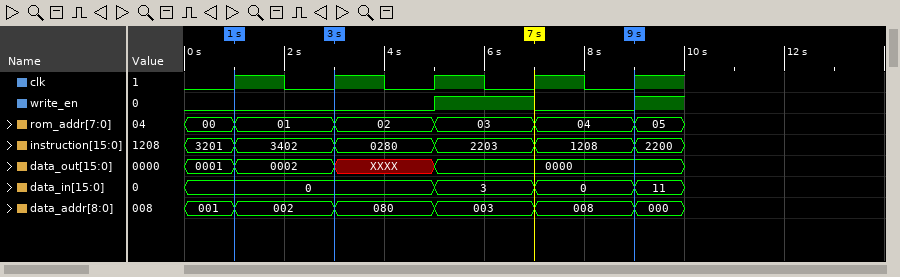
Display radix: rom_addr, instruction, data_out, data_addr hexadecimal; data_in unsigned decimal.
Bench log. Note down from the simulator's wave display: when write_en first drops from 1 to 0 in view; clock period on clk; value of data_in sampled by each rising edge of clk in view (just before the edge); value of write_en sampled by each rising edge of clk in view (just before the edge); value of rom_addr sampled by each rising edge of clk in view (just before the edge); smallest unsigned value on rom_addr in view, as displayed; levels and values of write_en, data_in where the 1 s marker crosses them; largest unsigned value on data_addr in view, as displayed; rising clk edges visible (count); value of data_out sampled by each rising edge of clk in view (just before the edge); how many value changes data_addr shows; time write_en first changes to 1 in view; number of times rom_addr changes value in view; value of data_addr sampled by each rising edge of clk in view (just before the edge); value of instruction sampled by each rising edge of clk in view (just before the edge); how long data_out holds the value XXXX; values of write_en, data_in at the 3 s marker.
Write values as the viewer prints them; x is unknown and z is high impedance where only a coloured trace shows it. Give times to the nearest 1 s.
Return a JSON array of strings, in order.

["7 s", "2 s", "0, 0, 0, 3, 0", "0 0 0 1 0", "00, 01, 02, 03, 04", "00", "write_en=0, data_in=0", "080", "5", "0001, 0002, XXXX, 0000, 0000", "5", "5 s", "5", "001, 002, 080, 003, 008", "3201, 3402, 0280, 2203, 1208", "2 s", "write_en=0, data_in=0"]
